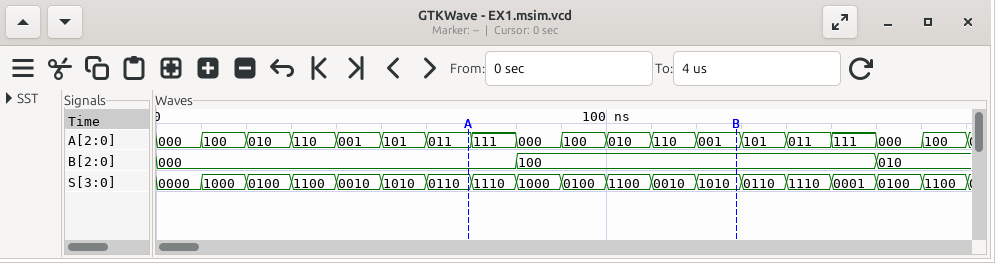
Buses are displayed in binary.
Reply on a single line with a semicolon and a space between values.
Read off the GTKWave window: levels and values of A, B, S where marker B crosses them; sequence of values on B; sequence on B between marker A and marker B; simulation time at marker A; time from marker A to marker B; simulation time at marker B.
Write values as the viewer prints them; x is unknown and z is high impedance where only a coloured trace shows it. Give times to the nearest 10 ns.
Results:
A=001, B=100, S=1010; 000, 100, 010; 000, 100; 70 ns; 60 ns; 130 ns
